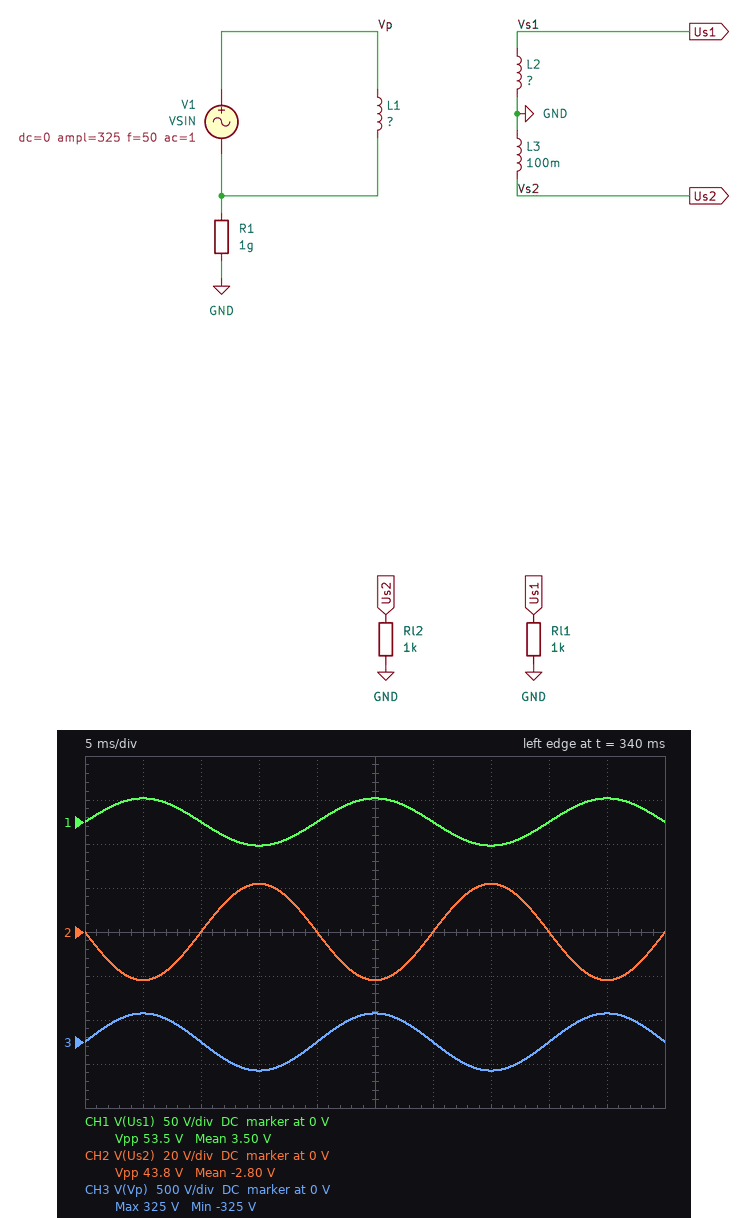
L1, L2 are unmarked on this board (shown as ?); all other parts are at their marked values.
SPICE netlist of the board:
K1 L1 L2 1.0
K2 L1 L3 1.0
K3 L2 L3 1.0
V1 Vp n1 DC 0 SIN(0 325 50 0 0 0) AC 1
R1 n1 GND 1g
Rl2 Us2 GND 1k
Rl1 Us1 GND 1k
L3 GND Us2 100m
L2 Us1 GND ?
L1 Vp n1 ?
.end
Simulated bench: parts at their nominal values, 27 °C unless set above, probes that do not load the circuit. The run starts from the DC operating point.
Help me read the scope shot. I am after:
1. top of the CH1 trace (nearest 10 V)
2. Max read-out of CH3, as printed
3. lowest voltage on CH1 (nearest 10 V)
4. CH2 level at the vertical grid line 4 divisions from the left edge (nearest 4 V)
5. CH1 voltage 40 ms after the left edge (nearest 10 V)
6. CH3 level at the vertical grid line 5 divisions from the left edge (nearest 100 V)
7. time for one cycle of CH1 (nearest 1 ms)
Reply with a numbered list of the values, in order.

1. 30 V
2. 325 V
3. -30 V
4. 0 V
5. 0 V
6. 300 V
7. 20 ms
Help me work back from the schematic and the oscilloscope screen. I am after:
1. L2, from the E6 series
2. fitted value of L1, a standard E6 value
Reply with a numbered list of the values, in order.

1. 150 mH
2. 22 H
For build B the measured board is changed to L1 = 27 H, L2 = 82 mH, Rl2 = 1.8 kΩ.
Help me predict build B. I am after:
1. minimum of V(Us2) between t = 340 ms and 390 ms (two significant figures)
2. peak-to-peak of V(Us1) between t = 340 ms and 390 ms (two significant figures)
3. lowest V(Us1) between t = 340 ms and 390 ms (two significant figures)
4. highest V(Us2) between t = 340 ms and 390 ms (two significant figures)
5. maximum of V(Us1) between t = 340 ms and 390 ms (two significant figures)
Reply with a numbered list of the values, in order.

1. -20 V
2. 36 V
3. -18 V
4. 20 V
5. 18 V
